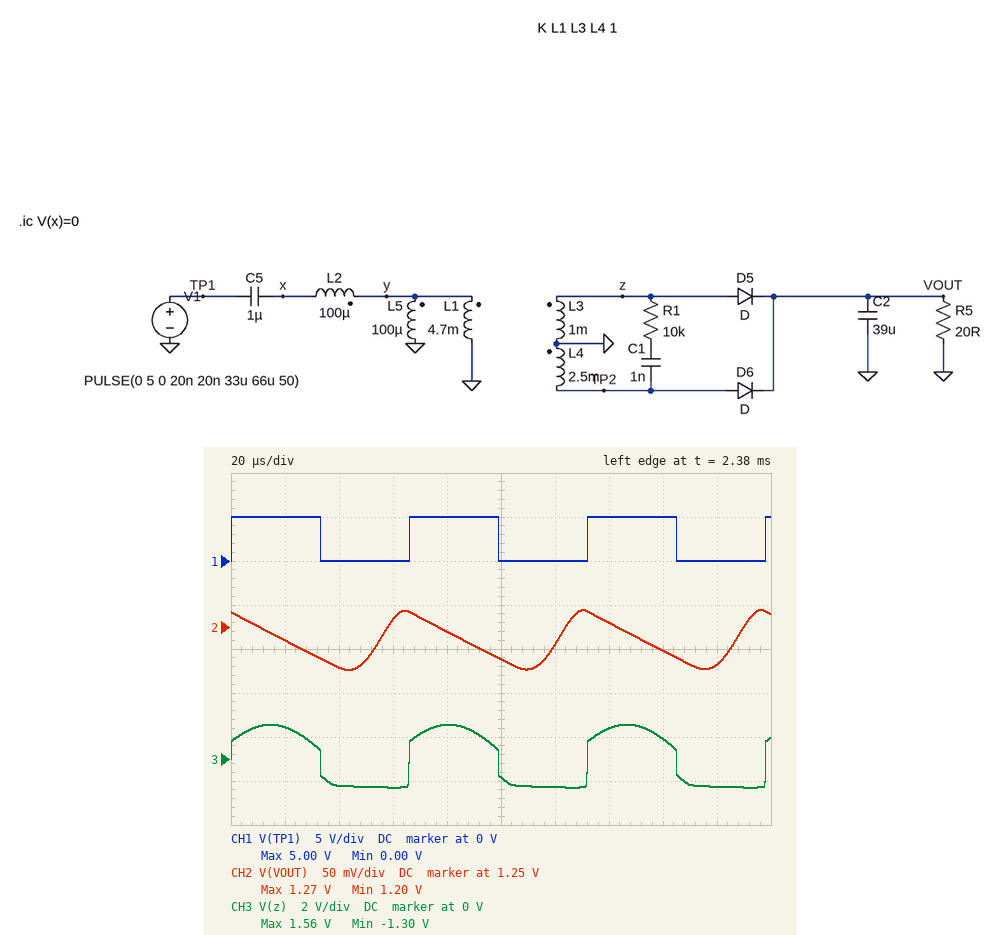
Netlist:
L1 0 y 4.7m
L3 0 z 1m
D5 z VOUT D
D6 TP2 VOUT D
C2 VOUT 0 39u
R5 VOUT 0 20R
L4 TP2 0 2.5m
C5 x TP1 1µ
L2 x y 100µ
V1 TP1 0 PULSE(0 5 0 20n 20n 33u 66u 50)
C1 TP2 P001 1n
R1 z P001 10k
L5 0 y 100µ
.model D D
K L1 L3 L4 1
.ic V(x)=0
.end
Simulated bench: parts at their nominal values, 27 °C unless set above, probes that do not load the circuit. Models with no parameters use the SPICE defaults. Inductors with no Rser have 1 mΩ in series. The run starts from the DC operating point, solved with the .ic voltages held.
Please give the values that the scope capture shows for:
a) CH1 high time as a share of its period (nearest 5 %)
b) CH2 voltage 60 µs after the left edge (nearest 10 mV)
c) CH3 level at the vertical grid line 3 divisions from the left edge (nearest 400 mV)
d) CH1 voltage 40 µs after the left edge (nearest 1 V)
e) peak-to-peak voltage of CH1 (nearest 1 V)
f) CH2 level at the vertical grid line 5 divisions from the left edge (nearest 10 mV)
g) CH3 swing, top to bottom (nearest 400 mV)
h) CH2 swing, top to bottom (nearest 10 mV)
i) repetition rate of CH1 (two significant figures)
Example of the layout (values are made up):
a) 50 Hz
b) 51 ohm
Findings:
a) 50 %
b) 1.26 V
c) -1.2 V
d) 0 V
e) 5 V
f) 1.21 V
g) 2.8 V
h) 70 mV
i) 15 kHz
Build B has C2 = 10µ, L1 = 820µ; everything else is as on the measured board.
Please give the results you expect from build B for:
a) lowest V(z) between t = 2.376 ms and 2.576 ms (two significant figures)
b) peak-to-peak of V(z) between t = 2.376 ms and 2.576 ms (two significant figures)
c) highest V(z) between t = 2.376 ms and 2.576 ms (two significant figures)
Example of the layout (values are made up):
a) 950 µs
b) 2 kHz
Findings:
a) -3.0 V
b) 7.6 V
c) 4.6 V
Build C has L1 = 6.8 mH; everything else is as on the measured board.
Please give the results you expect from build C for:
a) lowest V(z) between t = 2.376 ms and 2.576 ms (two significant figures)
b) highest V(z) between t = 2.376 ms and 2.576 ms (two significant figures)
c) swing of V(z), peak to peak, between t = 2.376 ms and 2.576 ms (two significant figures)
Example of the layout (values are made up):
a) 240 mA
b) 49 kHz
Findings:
a) -1.1 V
b) 1.3 V
c) 2.4 V
